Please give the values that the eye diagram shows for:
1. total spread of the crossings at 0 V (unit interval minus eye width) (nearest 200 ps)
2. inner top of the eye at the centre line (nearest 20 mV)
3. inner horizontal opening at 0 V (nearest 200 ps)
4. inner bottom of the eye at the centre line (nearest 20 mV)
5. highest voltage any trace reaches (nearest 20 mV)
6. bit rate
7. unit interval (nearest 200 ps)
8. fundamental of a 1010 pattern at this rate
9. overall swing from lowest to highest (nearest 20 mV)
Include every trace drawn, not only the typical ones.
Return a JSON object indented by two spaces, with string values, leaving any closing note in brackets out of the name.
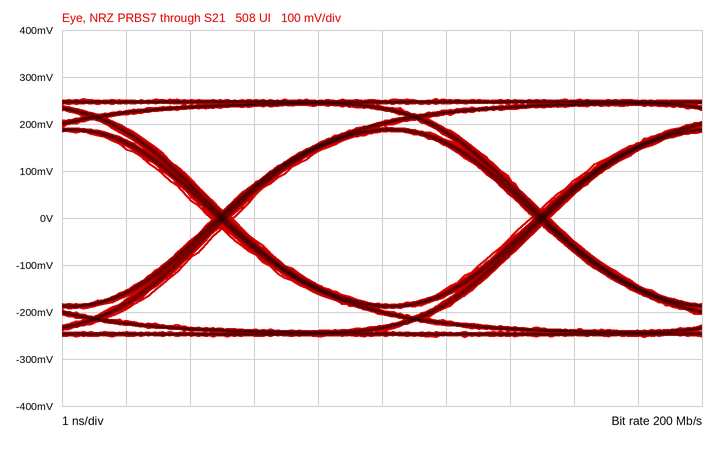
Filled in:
{
  "total spread of the crossings at 0 V (unit interval minus eye width)": "400 ps",
  "inner top of the eye at the centre line": "180 mV",
  "inner horizontal opening at 0 V": "4.6 ns",
  "inner bottom of the eye at the centre line": "-180 mV",
  "highest voltage any trace reaches": "260 mV",
  "bit rate": "200 Mb/s",
  "unit interval": "5.0 ns",
  "fundamental of a 1010 pattern at this rate": "100 MHz",
  "overall swing from lowest to highest": "500 mV"
}
